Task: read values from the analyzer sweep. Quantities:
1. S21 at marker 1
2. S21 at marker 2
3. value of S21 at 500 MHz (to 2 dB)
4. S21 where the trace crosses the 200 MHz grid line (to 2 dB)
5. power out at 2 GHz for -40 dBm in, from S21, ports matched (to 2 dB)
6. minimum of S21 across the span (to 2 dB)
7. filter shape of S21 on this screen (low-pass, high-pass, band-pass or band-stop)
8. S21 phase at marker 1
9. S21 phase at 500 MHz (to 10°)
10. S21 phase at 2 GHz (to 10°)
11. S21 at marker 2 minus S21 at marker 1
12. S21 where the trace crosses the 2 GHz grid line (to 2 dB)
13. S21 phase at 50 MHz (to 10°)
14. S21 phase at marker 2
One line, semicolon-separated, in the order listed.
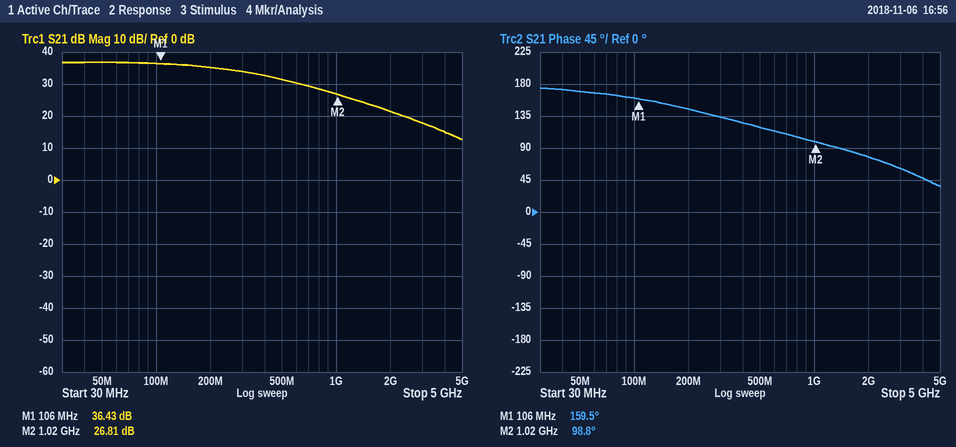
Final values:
36.43 dB; 26.81 dB; 32 dB; 36 dB; -18 dBm; 12 dB; low-pass; 159.5°; 120°; 80°; -9.62 dB; 22 dB; 170°; 98.8°
